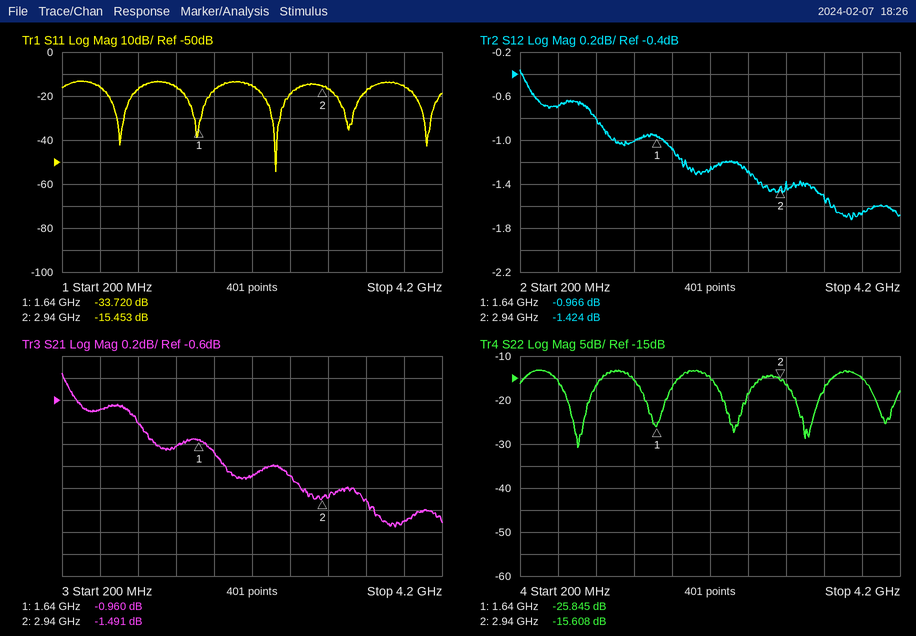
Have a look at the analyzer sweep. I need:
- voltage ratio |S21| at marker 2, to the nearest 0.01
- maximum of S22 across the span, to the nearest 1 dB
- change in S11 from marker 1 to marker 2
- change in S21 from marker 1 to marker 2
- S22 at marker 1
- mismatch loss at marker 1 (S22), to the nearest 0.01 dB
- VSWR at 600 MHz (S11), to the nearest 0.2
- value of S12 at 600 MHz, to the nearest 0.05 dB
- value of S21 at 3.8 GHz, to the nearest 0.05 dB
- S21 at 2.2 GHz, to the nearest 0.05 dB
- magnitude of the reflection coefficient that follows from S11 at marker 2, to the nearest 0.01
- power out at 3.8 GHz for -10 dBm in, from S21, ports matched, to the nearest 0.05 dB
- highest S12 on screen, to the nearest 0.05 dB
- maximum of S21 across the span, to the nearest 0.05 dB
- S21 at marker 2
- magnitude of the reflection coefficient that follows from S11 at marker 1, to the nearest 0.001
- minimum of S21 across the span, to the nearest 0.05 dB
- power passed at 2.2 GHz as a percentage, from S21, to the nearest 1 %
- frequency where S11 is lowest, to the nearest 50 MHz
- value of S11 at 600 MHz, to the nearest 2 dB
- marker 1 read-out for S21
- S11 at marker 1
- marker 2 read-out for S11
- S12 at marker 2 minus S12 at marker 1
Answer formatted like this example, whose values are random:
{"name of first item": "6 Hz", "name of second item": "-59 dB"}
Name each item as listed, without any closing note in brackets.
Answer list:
{"voltage ratio |S21| at marker 2, to the nearest 0.01": "0.84", "maximum of S22 across the span, to the nearest 1 dB": "-13 dB", "change in S11 from marker 1 to marker 2": "18.267 dB", "change in S21 from marker 1 to marker 2": "-0.531 dB", "S22 at marker 1": "-25.845 dB", "mismatch loss at marker 1 (S22), to the nearest 0.01 dB": "0.01 dB", "VSWR at 600 MHz (S11), to the nearest 0.2": "1.4", "value of S12 at 600 MHz, to the nearest 0.05 dB": "-0.70 dB", "value of S21 at 3.8 GHz, to the nearest 0.05 dB": "-1.70 dB", "S21 at 2.2 GHz, to the nearest 0.05 dB": "-1.30 dB", "magnitude of the reflection coefficient that follows from S11 at marker 2, to the nearest 0.01": "0.17", "power out at 3.8 GHz for -10 dBm in, from S21, ports matched, to the nearest 0.05 dB": "-11.70 dBm", "highest S12 on screen, to the nearest 0.05 dB": "-0.35 dB", "maximum of S21 across the span, to the nearest 0.05 dB": "-0.35 dB", "S21 at marker 2": "-1.491 dB", "magnitude of the reflection coefficient that follows from S11 at marker 1, to the nearest 0.001": "0.021", "minimum of S21 across the span, to the nearest 0.05 dB": "-1.75 dB", "power passed at 2.2 GHz as a percentage, from S21, to the nearest 1 %": "74 %", "frequency where S11 is lowest, to the nearest 50 MHz": "2.45 GHz", "value of S11 at 600 MHz, to the nearest 2 dB": "-16 dB", "marker 1 read-out for S21": "-0.960 dB", "S11 at marker 1": "-33.720 dB", "marker 2 read-out for S11": "-15.453 dB", "S12 at marker 2 minus S12 at marker 1": "-0.458 dB"}
